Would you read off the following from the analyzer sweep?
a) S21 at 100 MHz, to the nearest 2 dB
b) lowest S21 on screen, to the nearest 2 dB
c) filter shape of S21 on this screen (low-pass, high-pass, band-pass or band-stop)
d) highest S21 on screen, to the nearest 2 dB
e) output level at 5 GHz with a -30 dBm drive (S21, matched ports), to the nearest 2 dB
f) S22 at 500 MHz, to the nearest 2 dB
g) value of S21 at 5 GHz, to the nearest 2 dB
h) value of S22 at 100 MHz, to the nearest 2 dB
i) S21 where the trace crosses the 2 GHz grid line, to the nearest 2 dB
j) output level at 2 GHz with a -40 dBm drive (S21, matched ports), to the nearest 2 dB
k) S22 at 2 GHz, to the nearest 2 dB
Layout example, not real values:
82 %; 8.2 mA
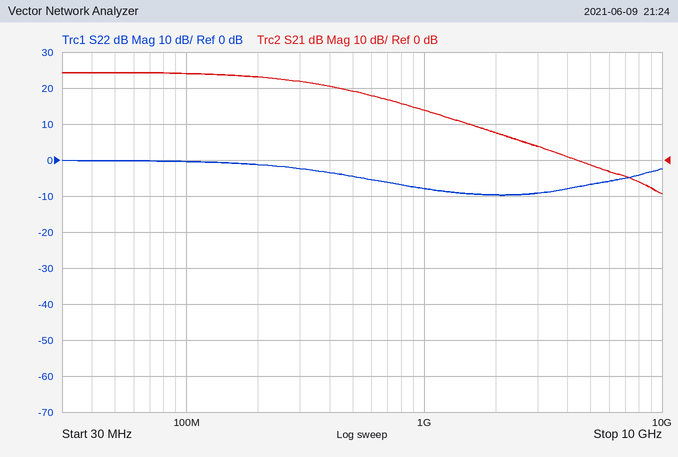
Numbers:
24 dB; -10 dB; low-pass; 24 dB; -32 dBm; -4 dB; -2 dB; 0 dB; 8 dB; -32 dBm; -10 dB
